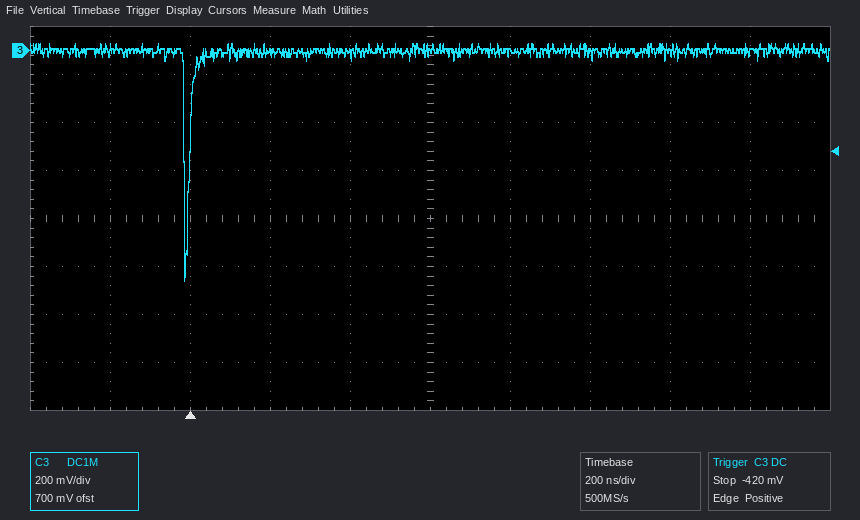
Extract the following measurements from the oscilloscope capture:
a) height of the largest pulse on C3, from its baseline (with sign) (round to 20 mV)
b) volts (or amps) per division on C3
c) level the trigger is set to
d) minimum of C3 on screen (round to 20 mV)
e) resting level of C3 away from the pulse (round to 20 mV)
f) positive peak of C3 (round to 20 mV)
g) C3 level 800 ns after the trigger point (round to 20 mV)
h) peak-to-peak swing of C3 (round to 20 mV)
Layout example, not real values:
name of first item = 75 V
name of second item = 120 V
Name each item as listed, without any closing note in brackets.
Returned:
height of the largest pulse on C3, from its baseline (with sign) = -960 mV
volts (or amps) per division on C3 = 200 mV
level the trigger is set to = -420 mV
minimum of C3 on screen = -960 mV
resting level of C3 away from the pulse = 0 mV
positive peak of C3 = 20 mV
C3 level 800 ns after the trigger point = 0 mV
peak-to-peak swing of C3 = 980 mV
